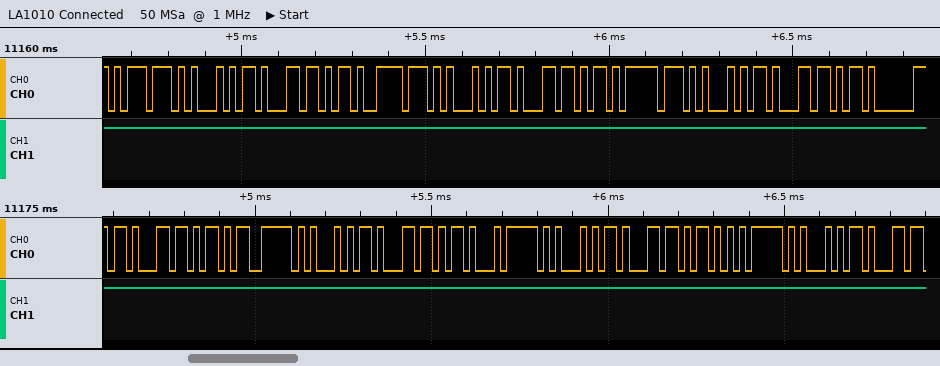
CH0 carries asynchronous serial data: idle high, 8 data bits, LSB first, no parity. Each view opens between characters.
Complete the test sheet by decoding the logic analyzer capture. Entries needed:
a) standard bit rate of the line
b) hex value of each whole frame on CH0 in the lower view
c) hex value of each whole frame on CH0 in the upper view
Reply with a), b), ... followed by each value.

a) 57600 baud
b) 8B, 6B, F3, 45, 8B, 6B, F4, 45, 8B, 6B, F5, 45, 8B
c) DD, 45, 8B, 6B, DE, 45, 8B, 6B, DF, 45, 8B, 6B
